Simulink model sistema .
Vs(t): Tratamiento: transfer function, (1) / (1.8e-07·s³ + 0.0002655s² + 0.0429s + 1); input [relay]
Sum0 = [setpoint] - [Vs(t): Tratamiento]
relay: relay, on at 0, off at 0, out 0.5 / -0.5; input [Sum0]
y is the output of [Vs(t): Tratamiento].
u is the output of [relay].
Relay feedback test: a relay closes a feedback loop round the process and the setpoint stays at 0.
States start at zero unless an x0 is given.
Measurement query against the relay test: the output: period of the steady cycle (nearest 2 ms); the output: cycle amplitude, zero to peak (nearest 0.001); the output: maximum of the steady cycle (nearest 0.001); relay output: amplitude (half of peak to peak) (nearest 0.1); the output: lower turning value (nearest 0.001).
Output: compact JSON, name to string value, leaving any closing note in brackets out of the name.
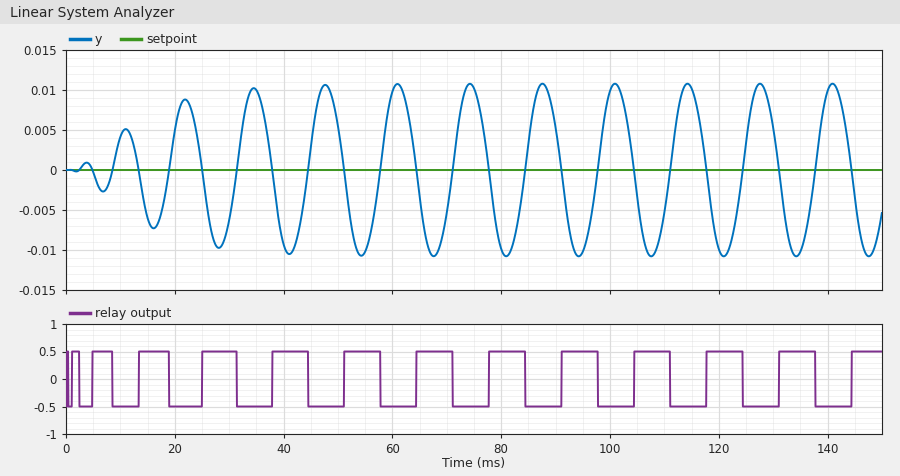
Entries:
{"the output: period of the steady cycle": "14 ms", "the output: cycle amplitude, zero to peak": "0.011", "the output: maximum of the steady cycle": "0.011", "relay output: amplitude (half of peak to peak)": "0.5", "the output: lower turning value": "-0.011"}
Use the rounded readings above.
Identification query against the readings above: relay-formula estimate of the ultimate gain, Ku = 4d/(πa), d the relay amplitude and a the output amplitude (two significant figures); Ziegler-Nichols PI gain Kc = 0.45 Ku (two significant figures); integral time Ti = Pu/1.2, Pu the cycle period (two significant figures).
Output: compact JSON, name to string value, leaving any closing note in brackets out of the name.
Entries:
{"relay-formula estimate of the ultimate gain, Ku = 4d/(πa), d the relay amplitude and a the output amplitude": "58", "Ziegler-Nichols PI gain Kc = 0.45 Ku": "26", "integral time Ti = Pu/1.2, Pu the cycle period": "12 ms"}
